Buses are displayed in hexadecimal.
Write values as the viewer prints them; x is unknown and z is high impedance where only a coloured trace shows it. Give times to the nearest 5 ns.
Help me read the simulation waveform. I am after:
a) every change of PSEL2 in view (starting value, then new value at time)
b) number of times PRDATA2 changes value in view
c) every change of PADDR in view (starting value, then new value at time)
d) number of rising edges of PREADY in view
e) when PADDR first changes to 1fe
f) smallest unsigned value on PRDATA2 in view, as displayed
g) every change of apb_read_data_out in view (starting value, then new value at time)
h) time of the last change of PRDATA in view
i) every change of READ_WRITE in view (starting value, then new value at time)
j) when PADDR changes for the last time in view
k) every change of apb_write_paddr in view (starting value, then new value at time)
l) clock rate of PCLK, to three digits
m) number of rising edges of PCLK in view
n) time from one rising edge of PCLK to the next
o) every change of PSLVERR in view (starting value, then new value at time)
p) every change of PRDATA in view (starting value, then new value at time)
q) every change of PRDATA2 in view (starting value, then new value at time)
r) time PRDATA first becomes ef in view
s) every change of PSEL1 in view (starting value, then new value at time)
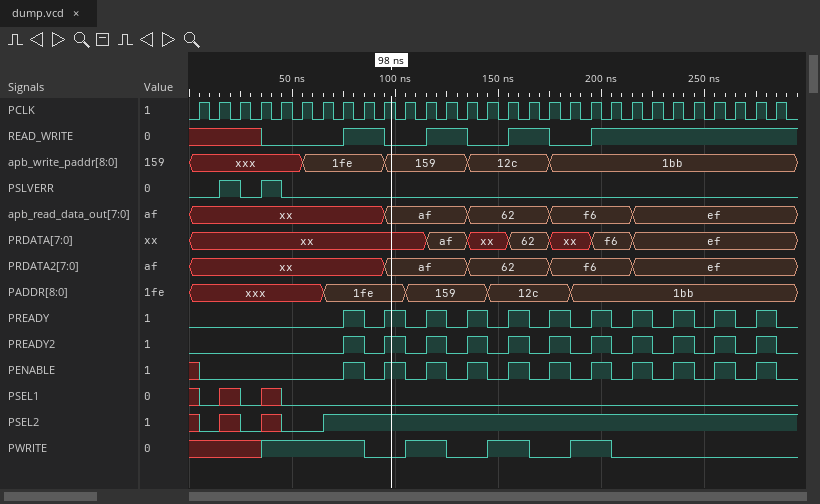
x, 0 at 5 ns, x at 15 ns, 0 at 25 ns, x at 35 ns, 0 at 45 ns, 1 at 65 ns
4
xxx, 1fe at 65 ns, 159 at 105 ns, 12c at 145 ns, 1bb at 185 ns
11
65 ns
62
xx, af at 95 ns, 62 at 135 ns, f6 at 175 ns, ef at 215 ns
215 ns
x, 0 at 35 ns, 1 at 75 ns, 0 at 95 ns, 1 at 115 ns, 0 at 135 ns, 1 at 155 ns, 0 at 175 ns, 1 at 195 ns
185 ns
xxx, 1fe at 55 ns, 159 at 95 ns, 12c at 135 ns, 1bb at 175 ns
100 MHz
29
10 ns
0, 1 at 15 ns, 0 at 25 ns, 1 at 35 ns, 0 at 45 ns
xx, af at 115 ns, xx at 135 ns, 62 at 155 ns, xx at 175 ns, f6 at 195 ns, ef at 215 ns
xx, af at 95 ns, 62 at 135 ns, f6 at 175 ns, ef at 215 ns
215 ns
x, 0 at 5 ns, x at 15 ns, 0 at 25 ns, x at 35 ns, 0 at 45 ns
